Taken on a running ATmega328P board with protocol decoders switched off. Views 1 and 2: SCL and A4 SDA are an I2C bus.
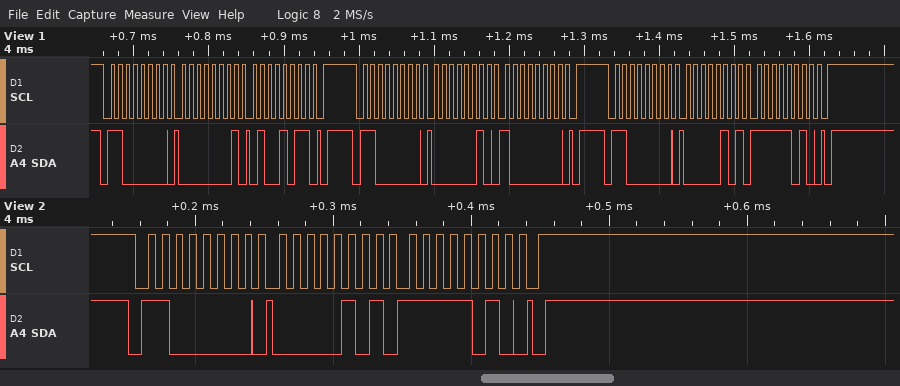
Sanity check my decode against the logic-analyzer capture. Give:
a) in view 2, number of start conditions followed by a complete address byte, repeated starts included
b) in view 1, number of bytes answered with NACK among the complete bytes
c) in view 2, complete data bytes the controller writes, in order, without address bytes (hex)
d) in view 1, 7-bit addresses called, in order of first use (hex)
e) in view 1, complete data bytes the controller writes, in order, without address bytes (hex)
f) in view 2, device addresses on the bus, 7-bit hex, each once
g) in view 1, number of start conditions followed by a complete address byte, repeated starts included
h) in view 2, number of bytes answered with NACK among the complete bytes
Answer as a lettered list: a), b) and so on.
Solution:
a) 1
b) 0
c) 05 FA
d) 0x60
e) 01 4B 02 80 05 FA
f) 0x60
g) 3
h) 0
